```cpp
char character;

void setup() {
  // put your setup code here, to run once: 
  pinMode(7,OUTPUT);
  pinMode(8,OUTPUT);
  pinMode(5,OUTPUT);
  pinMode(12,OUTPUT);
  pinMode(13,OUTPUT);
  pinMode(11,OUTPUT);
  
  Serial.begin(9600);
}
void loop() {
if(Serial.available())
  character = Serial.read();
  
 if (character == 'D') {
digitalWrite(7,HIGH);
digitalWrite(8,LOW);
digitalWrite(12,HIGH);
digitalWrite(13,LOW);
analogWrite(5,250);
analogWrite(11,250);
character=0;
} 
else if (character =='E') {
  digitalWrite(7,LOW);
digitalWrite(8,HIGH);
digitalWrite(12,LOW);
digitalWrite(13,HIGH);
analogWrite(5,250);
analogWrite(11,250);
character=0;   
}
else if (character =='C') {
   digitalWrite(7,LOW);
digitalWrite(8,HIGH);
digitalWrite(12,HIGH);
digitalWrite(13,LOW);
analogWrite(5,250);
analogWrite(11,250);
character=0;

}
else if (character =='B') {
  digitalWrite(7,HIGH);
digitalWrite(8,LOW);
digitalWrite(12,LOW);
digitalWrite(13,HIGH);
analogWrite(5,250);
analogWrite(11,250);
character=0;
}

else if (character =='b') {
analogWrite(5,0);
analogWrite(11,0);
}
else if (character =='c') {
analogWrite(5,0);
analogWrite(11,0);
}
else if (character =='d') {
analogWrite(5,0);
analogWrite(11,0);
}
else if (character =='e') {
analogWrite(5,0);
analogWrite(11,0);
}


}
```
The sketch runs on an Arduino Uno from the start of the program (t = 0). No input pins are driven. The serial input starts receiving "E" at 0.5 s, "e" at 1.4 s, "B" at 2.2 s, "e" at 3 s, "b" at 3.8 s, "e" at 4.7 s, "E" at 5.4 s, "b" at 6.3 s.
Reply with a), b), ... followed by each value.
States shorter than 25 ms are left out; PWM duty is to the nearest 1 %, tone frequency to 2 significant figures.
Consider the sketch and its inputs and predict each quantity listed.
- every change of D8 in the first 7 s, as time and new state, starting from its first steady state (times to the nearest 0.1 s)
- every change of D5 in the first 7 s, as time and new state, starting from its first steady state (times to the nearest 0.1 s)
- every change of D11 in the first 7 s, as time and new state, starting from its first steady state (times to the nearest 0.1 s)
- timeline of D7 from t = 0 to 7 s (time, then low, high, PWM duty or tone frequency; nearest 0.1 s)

a) 0 s low; 0.5 s high; 2.2 s low; 5.4 s high
b) 0 s low; 0.5 s PWM 98 %; 1.4 s low; 2.2 s PWM 98 %; 3 s low; 5.4 s PWM 98 %; 6.3 s low
c) 0 s low; 0.5 s PWM 98 %; 1.4 s low; 2.2 s PWM 98 %; 3 s low; 5.4 s PWM 98 %; 6.3 s low
d) 0 s low; 2.2 s high; 5.4 s low
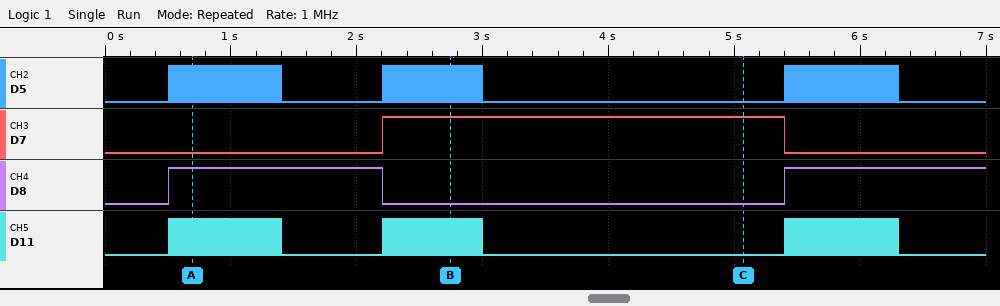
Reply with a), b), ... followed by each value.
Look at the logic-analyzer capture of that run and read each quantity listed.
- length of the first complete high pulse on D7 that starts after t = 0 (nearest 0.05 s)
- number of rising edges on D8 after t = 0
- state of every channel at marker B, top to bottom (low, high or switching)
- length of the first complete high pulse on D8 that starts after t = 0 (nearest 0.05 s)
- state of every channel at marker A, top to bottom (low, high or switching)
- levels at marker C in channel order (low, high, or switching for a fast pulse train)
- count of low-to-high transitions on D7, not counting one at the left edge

a) 3.20 s
b) 2
c) D5 switching, D7 high, D8 low, D11 switching
d) 1.70 s
e) D5 switching, D7 low, D8 high, D11 switching
f) D5 low, D7 high, D8 low, D11 low
g) 1
